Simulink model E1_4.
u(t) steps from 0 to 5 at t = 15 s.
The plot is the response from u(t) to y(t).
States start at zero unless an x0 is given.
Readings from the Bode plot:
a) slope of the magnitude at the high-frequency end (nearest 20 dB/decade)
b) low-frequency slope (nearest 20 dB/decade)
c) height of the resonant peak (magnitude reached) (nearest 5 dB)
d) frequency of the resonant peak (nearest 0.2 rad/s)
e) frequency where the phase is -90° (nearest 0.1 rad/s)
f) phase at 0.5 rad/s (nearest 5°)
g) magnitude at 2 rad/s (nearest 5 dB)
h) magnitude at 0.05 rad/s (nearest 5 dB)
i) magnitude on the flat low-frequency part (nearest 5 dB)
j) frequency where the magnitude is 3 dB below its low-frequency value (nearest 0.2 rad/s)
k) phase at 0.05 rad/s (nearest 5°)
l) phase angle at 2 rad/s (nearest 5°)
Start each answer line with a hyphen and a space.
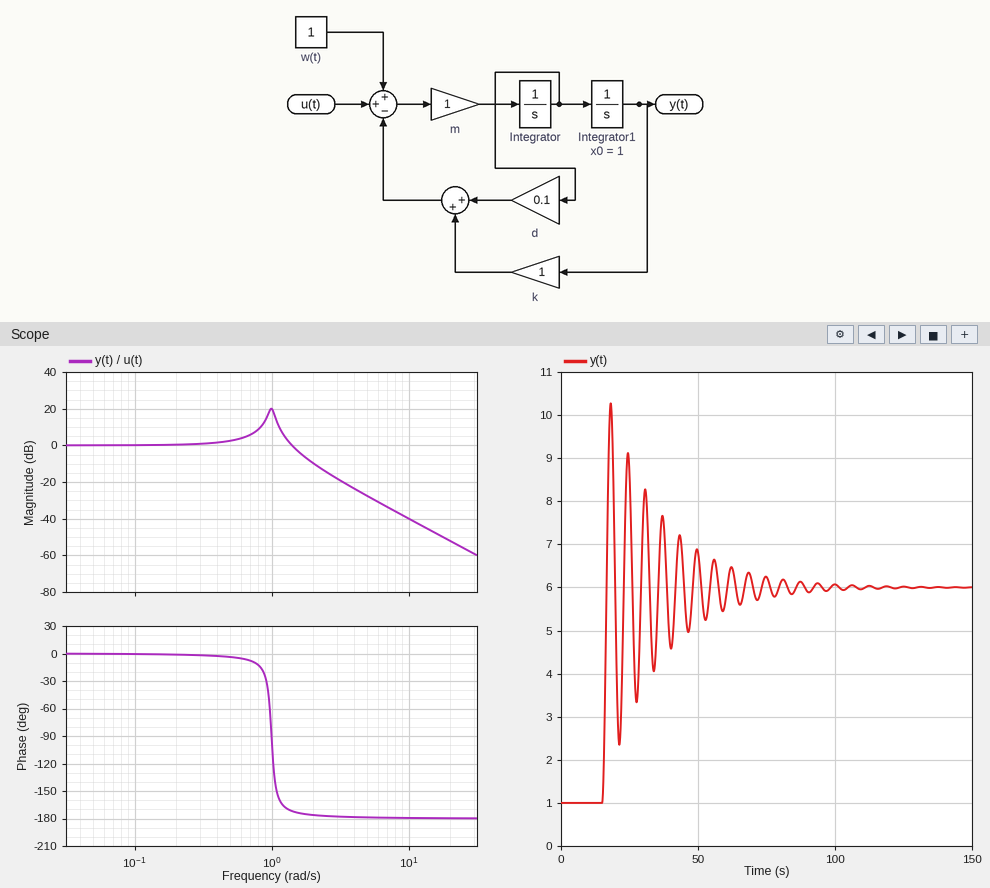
- -40 dB/decade
- 0 dB/decade
- 20 dB
- 1.0 rad/s
- 1.0 rad/s
- -5°
- -10 dB
- 0 dB
- 0 dB
- 1.6 rad/s
- 0°
- -175°
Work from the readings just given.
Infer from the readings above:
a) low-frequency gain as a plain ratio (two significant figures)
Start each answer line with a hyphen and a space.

- 1.0
